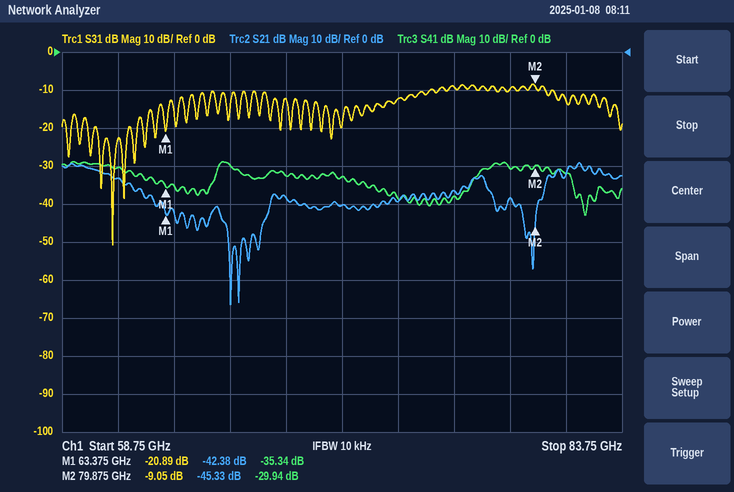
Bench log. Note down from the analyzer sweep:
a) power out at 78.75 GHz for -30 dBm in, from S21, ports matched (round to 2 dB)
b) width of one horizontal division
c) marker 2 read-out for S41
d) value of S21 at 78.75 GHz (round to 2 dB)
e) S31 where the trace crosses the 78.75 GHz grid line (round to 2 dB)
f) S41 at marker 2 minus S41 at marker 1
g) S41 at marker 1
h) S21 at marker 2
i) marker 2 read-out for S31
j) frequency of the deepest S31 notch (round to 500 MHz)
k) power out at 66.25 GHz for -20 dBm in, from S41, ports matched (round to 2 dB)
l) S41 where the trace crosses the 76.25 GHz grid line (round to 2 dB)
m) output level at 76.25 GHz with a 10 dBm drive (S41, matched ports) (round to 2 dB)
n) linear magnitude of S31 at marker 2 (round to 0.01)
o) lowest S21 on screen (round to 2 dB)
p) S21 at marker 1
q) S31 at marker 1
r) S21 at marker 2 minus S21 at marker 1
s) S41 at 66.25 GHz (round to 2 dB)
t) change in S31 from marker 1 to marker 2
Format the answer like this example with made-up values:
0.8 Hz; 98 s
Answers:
-68 dBm; 2.5 GHz; -29.94 dB; -38 dB; -10 dB; 5.40 dB; -35.34 dB; -45.33 dB; -9.05 dB; 61.0 GHz; -50 dBm; -38 dB; -28 dBm; 0.35; -66 dB; -42.38 dB; -20.89 dB; -2.95 dB; -30 dB; 11.84 dB
